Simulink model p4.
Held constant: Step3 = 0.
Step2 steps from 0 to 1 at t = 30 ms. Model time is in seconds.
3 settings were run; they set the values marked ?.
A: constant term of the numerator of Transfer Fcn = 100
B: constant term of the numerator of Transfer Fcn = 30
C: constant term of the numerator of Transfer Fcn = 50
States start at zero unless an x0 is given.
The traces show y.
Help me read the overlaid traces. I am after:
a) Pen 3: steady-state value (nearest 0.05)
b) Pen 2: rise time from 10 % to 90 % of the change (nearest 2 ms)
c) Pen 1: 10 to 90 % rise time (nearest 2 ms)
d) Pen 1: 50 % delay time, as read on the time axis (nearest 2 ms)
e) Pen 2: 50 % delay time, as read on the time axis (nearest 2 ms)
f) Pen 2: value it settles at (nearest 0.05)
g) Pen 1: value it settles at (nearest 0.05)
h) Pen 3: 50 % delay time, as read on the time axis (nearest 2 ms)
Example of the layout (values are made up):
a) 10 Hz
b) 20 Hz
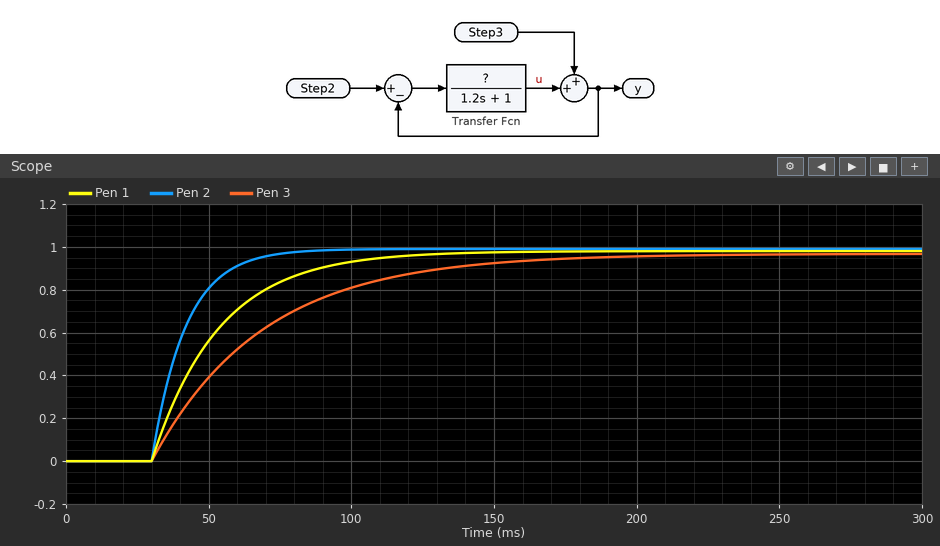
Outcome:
a) 0.95
b) 26 ms
c) 52 ms
d) 46 ms
e) 38 ms
f) 1.00
g) 1.00
h) 56 ms
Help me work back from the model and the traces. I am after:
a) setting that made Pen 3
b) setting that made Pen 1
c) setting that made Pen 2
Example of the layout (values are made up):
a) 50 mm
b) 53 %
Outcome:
a) B
b) C
c) A
